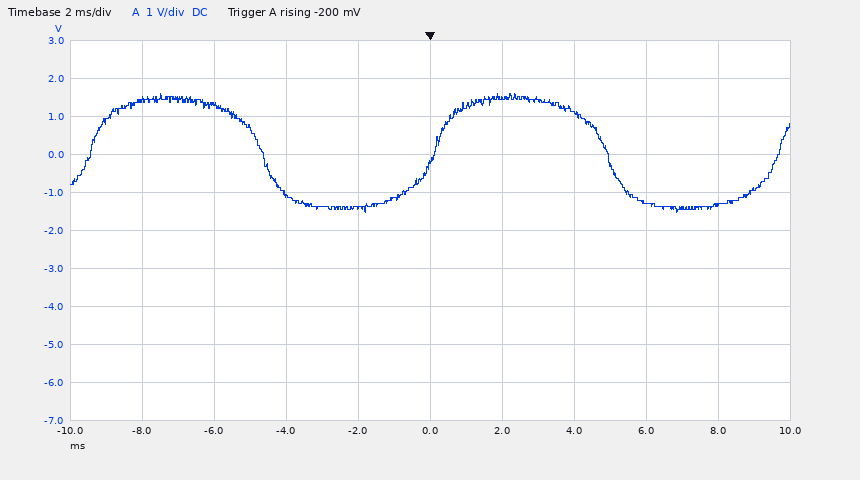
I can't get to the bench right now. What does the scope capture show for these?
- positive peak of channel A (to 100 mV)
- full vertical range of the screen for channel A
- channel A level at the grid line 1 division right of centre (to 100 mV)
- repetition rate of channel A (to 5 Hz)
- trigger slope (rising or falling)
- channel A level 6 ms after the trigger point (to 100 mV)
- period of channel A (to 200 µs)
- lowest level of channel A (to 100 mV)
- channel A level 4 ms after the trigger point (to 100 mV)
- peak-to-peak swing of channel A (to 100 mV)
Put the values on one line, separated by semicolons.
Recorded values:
1.6 V; 10 V; 1.5 V; 105 Hz; rising; -1.2 V; 9.6 ms; -1.5 V; 1.1 V; 3.1 V
